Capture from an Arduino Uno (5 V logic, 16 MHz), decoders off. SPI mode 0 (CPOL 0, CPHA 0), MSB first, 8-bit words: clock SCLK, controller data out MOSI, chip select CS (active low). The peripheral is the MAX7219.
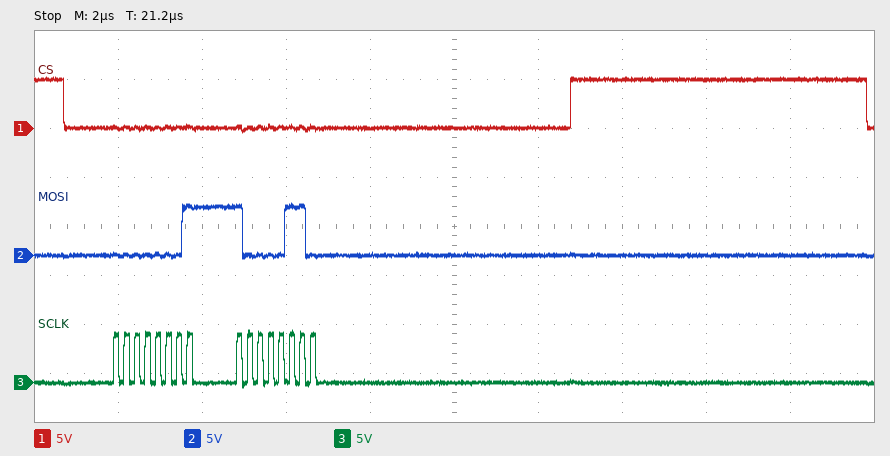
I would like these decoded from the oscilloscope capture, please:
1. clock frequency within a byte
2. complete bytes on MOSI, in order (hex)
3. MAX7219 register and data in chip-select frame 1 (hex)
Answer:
4 MHz
01 86
register 0x1, data 0x86
